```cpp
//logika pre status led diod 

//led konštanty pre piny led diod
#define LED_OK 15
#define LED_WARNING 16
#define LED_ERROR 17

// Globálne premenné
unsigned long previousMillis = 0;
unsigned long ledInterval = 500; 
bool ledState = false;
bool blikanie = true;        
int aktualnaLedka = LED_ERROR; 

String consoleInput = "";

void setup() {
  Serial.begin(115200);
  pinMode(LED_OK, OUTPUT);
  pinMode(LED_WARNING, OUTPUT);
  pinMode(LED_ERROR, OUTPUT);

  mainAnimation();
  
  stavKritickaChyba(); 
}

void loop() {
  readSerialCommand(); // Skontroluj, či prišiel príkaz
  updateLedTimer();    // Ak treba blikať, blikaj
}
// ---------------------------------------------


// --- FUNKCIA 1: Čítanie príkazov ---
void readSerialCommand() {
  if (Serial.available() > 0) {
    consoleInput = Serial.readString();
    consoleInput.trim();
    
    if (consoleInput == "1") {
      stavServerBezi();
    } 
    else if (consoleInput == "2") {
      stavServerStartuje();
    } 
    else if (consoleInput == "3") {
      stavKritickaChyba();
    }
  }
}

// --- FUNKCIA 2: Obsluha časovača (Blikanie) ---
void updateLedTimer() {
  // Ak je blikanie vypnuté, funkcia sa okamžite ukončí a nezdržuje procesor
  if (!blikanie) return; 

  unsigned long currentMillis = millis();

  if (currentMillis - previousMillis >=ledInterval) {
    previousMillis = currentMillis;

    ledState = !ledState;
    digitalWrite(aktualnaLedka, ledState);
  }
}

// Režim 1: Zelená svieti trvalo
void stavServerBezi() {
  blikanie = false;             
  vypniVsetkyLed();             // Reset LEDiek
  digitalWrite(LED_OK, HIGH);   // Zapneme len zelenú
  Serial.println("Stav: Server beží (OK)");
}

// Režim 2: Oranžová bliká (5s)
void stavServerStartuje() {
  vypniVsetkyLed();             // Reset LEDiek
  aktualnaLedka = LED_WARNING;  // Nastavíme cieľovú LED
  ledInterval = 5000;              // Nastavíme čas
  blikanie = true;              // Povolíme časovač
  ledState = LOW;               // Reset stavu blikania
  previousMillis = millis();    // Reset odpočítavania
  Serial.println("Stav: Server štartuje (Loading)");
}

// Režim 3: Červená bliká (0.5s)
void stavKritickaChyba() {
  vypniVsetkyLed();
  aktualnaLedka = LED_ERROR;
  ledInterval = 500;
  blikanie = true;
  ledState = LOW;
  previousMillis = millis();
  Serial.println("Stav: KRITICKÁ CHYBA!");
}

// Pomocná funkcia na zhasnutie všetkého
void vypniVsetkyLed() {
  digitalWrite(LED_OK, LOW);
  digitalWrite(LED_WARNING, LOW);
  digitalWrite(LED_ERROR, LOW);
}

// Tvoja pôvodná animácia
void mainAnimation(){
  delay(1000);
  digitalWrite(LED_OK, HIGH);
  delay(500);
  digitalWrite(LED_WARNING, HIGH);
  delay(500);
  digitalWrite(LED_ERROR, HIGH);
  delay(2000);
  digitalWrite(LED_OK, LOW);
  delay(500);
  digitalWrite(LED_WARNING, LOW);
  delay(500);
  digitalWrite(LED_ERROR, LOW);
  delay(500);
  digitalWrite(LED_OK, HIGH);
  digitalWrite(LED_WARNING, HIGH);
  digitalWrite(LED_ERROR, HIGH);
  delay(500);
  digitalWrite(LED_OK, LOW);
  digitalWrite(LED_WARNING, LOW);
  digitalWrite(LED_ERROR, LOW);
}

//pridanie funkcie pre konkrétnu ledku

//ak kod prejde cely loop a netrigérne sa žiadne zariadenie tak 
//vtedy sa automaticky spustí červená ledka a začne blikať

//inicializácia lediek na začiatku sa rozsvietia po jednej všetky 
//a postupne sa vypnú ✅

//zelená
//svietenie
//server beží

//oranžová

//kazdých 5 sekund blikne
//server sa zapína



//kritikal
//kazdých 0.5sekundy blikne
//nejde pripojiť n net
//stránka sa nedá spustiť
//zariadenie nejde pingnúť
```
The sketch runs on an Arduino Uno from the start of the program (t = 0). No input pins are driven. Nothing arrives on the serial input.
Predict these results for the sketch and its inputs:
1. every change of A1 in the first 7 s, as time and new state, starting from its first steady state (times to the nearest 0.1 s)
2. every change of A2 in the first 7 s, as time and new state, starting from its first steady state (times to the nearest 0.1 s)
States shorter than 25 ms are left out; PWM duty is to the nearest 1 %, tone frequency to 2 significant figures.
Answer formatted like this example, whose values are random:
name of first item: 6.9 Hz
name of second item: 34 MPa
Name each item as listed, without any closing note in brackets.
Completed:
every change of A1 in the first 7 s, as time and new state, starting from its first steady state: 0 s low; 1 s high; 4 s low; 5.5 s high; 6 s low
every change of A2 in the first 7 s, as time and new state, starting from its first steady state: 0 s low; 1.5 s high; 4.5 s low; 5.5 s high; 6 s low
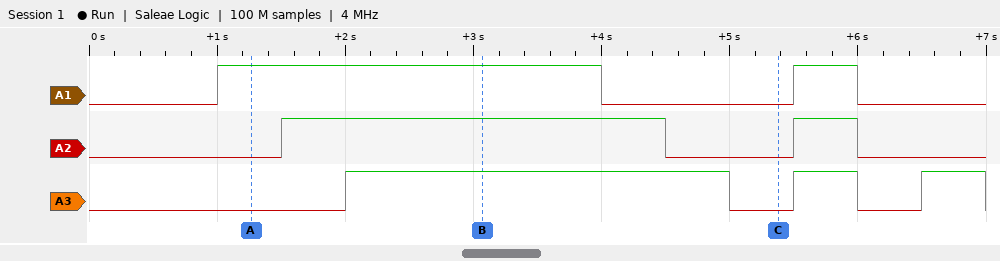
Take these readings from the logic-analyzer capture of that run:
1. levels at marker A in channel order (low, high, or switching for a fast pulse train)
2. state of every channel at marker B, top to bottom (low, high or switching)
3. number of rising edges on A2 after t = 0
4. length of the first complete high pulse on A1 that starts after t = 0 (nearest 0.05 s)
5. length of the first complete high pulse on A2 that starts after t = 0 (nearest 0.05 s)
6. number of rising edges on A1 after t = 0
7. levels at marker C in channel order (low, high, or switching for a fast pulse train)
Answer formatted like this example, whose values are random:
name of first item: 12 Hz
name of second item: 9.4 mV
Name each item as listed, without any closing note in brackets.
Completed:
levels at marker A in channel order: A1 high, A2 low, A3 low
state of every channel at marker B, top to bottom: A1 high, A2 high, A3 high
number of rising edges on A2 after t = 0: 2
length of the first complete high pulse on A1 that starts after t = 0: 3.00 s
length of the first complete high pulse on A2 that starts after t = 0: 3.00 s
number of rising edges on A1 after t = 0: 2
levels at marker C in channel order: A1 low, A2 low, A3 low
